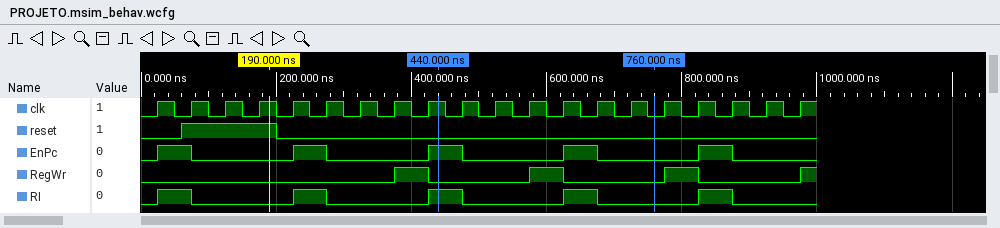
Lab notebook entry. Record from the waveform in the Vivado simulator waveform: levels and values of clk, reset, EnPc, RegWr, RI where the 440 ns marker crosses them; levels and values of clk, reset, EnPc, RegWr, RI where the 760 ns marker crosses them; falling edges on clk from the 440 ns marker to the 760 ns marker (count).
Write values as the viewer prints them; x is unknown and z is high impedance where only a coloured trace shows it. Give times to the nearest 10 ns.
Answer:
clk=1, reset=0, EnPc=1, RegWr=0, RI=1
clk=0, reset=0, EnPc=0, RegWr=0, RI=0
7
